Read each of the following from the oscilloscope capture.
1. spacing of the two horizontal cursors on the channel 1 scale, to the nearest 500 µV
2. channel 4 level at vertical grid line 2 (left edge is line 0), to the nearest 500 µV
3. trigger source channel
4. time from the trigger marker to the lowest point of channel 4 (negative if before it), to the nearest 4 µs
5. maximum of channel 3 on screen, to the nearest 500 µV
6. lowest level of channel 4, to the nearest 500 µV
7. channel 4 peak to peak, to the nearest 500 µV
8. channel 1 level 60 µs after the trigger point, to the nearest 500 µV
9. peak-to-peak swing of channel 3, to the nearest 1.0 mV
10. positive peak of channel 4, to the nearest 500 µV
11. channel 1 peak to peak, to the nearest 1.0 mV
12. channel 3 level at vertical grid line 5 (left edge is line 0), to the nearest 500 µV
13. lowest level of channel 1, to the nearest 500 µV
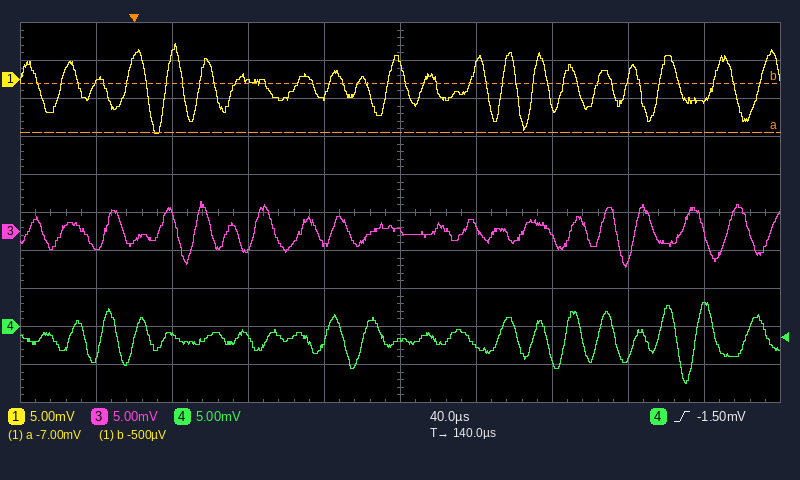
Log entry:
6.5 mV
-1.0 mV
channel 4
+292 µs
4.0 mV
-7.5 mV
10.5 mV
0.0 mV
9.0 mV
3.0 mV
12.0 mV
0.0 mV
-7.0 mV
